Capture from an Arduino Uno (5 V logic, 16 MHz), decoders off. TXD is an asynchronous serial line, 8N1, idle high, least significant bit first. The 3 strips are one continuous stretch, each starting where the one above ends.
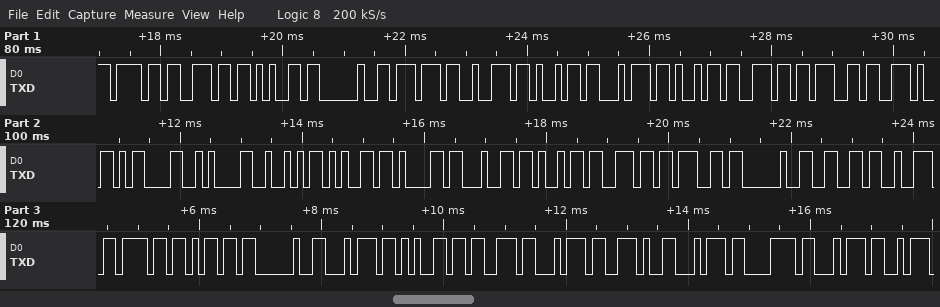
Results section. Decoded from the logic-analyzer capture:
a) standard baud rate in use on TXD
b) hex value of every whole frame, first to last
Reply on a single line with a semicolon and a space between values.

9600 baud; 6F 6E 65 20 77 72 69 74 69 6E 67 2E 0D 0A 52 65 61 64 69 6E 67 20 66 72 6F 6D 20 74 65 73 74 2E 74 78 74
